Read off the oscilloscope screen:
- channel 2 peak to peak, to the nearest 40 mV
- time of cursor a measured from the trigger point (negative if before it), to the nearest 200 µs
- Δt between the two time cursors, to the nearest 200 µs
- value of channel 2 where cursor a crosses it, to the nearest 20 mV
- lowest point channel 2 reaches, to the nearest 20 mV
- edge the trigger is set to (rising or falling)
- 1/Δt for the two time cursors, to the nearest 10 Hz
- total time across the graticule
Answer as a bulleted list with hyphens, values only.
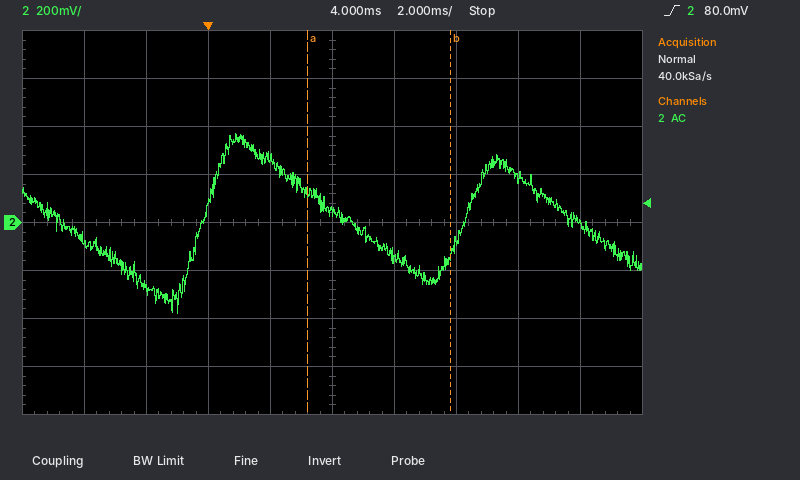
- 760 mV
- +3.2 ms
- 4.6 ms
- 120 mV
- -380 mV
- rising
- 220 Hz
- 20 ms
